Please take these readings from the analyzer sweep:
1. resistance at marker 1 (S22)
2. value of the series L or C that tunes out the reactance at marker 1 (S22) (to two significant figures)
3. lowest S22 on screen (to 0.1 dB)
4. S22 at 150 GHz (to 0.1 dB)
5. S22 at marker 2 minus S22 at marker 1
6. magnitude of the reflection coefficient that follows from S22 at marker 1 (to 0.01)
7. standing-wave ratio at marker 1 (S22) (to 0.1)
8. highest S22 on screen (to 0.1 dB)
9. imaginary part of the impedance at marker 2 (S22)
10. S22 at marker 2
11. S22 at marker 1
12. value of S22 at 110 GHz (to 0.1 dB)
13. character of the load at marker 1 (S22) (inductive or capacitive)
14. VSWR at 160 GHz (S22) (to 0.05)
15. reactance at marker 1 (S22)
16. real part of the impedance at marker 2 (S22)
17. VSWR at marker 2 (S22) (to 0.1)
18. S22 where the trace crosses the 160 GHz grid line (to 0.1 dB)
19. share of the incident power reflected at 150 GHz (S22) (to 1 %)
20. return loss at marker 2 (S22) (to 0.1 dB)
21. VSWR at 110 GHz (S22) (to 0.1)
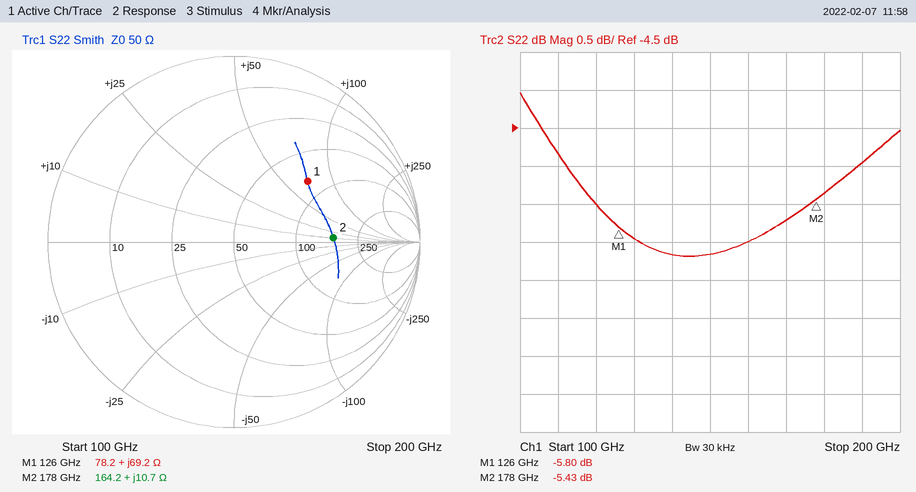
78.2 Ω
18 fF
-6.2 dB
-6.2 dB
0.37 dB
0.51
3.1
-4.0 dB
+10.7 Ω
-5.43 dB
-5.80 dB
-4.8 dB
inductive
3.00
+69.2 Ω
164.2 Ω
3.3
-6.0 dB
24 %
5.4 dB
3.7
